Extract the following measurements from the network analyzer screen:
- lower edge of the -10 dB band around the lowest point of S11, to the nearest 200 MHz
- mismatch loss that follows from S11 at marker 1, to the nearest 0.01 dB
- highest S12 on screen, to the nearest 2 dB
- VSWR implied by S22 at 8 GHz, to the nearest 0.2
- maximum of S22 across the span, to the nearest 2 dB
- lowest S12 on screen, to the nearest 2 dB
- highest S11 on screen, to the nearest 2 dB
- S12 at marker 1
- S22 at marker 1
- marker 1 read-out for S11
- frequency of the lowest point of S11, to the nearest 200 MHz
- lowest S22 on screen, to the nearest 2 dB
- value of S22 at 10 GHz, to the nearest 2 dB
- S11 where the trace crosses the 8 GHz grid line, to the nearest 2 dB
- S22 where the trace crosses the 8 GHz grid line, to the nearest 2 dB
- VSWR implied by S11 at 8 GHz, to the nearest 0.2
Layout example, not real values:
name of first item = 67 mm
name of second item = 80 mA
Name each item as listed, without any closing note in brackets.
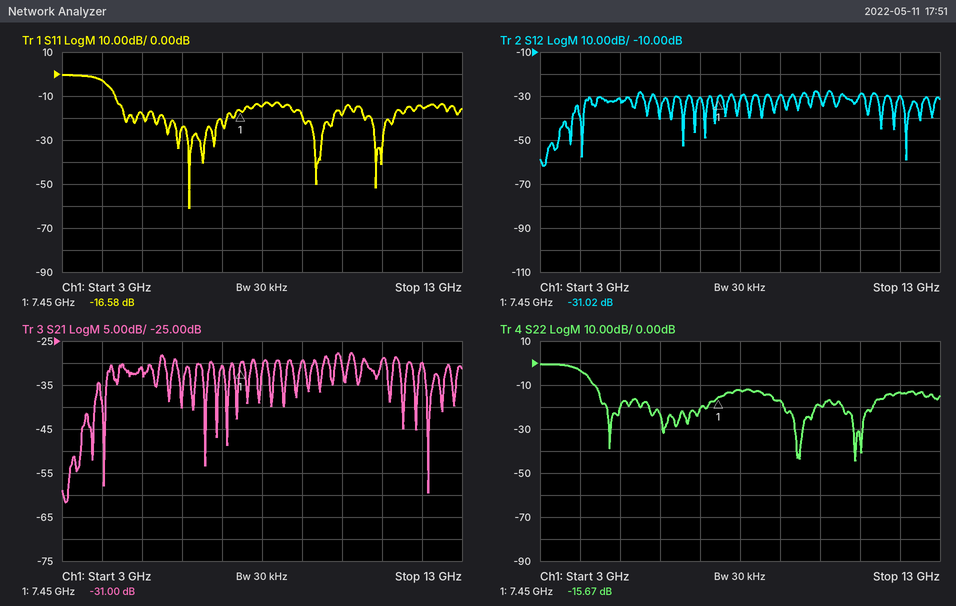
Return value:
lower edge of the -10 dB band around the lowest point of S11, to the nearest 200 MHz = 4.4 GHz
mismatch loss that follows from S11 at marker 1, to the nearest 0.01 dB = 0.10 dB
highest S12 on screen, to the nearest 2 dB = -28 dB
VSWR implied by S22 at 8 GHz, to the nearest 0.2 = 1.6
maximum of S22 across the span, to the nearest 2 dB = 0 dB
lowest S12 on screen, to the nearest 2 dB = -62 dB
highest S11 on screen, to the nearest 2 dB = 0 dB
S12 at marker 1 = -31.02 dB
S22 at marker 1 = -15.67 dB
marker 1 read-out for S11 = -16.58 dB
frequency of the lowest point of S11, to the nearest 200 MHz = 6.2 GHz
lowest S22 on screen, to the nearest 2 dB = -44 dB
value of S22 at 10 GHz, to the nearest 2 dB = -20 dB
S11 where the trace crosses the 8 GHz grid line, to the nearest 2 dB = -14 dB
S22 where the trace crosses the 8 GHz grid line, to the nearest 2 dB = -12 dB
VSWR implied by S11 at 8 GHz, to the nearest 0.2 = 1.4
